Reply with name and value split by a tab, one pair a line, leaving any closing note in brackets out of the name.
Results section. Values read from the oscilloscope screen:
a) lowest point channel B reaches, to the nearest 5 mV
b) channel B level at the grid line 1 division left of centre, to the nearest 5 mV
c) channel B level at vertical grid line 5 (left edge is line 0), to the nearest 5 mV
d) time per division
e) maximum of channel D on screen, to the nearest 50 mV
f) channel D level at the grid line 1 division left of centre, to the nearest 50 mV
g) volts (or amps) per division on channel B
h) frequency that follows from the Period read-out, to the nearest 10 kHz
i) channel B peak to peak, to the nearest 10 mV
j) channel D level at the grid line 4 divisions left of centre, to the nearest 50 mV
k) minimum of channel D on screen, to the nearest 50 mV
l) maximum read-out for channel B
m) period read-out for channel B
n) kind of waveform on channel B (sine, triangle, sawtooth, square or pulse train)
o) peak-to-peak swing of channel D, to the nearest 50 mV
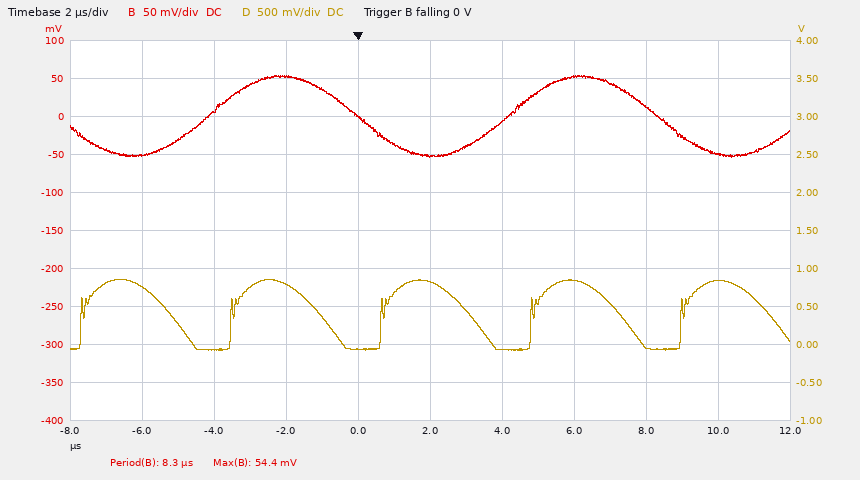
lowest point channel B reaches, to the nearest 5 mV	-55 mV
channel B level at the grid line 1 division left of centre, to the nearest 5 mV	0 mV
channel B level at vertical grid line 5 (left edge is line 0), to the nearest 5 mV	-50 mV
time per division	2 µs
maximum of channel D on screen, to the nearest 50 mV	850 mV
channel D level at the grid line 1 division left of centre, to the nearest 50 mV	-50 mV
volts (or amps) per division on channel B	50 mV
frequency that follows from the Period read-out, to the nearest 10 kHz	120 kHz
channel B peak to peak, to the nearest 10 mV	110 mV
channel D level at the grid line 4 divisions left of centre, to the nearest 50 mV	750 mV
minimum of channel D on screen, to the nearest 50 mV	-100 mV
maximum read-out for channel B	54.4 mV
period read-out for channel B	8.3 µs
kind of waveform on channel B	sine
peak-to-peak swing of channel D, to the nearest 50 mV	950 mV
